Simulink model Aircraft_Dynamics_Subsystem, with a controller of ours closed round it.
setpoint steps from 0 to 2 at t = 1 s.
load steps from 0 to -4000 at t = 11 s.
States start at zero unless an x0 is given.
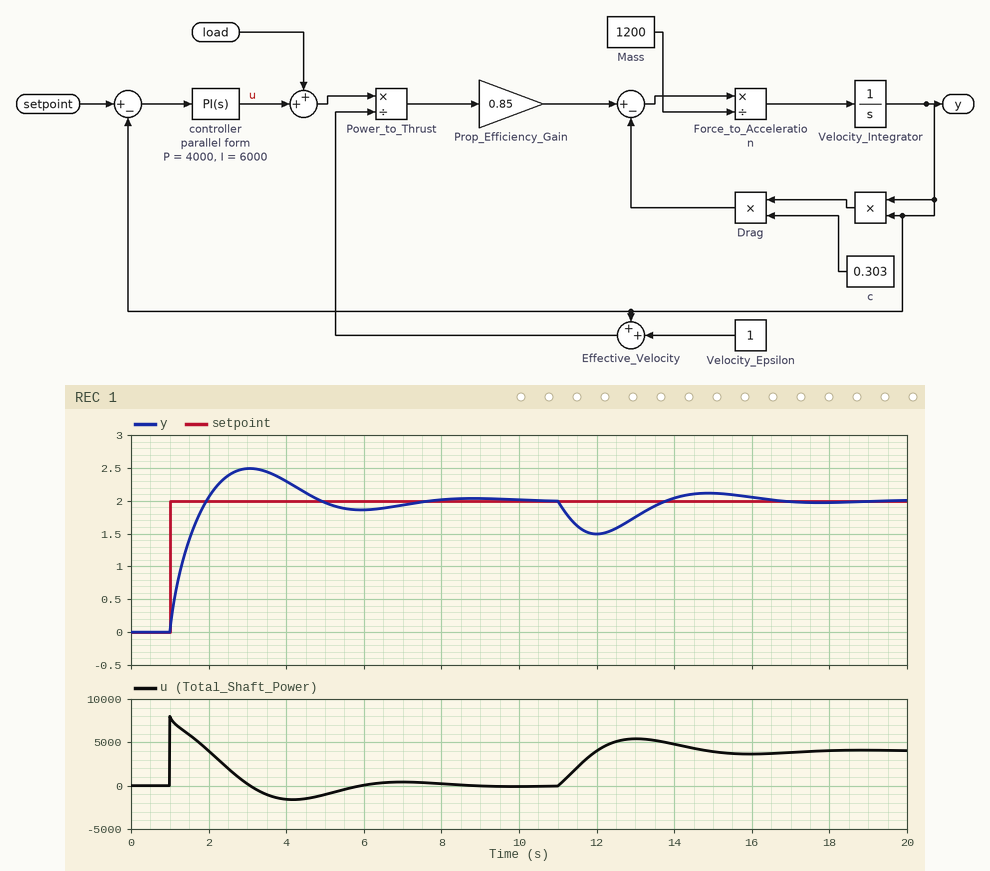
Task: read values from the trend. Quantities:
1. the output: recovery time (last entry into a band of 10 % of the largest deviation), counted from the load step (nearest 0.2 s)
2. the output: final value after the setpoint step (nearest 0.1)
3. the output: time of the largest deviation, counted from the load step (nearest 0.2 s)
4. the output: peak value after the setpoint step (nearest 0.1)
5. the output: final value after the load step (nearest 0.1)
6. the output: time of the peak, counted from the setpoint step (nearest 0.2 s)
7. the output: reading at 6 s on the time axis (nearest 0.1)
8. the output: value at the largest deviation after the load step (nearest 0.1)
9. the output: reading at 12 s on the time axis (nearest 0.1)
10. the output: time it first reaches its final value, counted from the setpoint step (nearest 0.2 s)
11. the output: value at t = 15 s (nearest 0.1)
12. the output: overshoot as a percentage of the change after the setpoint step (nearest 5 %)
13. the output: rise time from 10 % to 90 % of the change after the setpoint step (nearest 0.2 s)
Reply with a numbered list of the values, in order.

1. 5.0 s
2. 2.0
3. 1.0 s
4. 2.5
5. 2.0
6. 2.0 s
7. 1.9
8. 1.5
9. 1.5
10. 1.0 s
11. 2.1
12. 25 %
13. 0.8 s
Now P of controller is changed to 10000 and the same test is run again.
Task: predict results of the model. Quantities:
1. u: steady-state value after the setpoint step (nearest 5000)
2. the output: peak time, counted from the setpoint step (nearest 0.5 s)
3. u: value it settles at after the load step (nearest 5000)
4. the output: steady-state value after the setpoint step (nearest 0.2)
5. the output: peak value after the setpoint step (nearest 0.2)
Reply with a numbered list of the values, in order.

1. 0
2. 1.5 s
3. 5000
4. 2.0
5. 2.2
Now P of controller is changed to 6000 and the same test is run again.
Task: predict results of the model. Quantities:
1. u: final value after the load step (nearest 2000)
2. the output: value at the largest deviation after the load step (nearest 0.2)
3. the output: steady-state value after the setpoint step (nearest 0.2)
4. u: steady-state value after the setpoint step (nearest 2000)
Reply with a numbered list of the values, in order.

1. 4000
2. 1.6
3. 2.0
4. 0
